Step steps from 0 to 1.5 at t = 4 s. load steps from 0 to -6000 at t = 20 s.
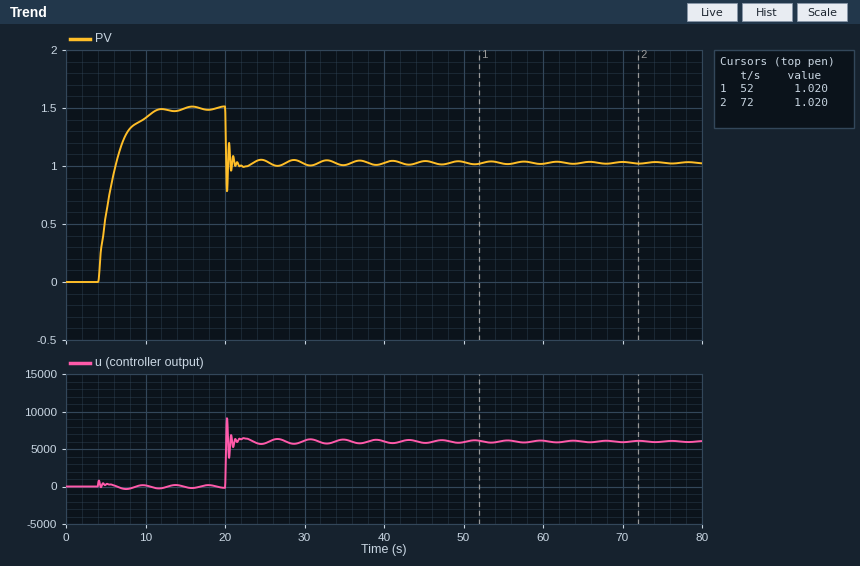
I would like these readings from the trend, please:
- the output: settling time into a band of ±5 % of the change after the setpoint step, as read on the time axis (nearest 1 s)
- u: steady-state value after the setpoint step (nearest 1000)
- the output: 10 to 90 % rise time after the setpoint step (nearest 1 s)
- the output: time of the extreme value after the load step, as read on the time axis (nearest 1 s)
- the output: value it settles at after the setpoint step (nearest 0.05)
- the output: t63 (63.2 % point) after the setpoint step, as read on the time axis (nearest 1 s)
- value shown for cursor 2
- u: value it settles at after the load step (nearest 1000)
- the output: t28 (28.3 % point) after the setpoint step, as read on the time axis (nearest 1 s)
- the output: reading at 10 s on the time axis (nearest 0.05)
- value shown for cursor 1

10 s
0
4 s
20 s
1.50
6 s
1.020
6000
5 s
1.40
1.020
